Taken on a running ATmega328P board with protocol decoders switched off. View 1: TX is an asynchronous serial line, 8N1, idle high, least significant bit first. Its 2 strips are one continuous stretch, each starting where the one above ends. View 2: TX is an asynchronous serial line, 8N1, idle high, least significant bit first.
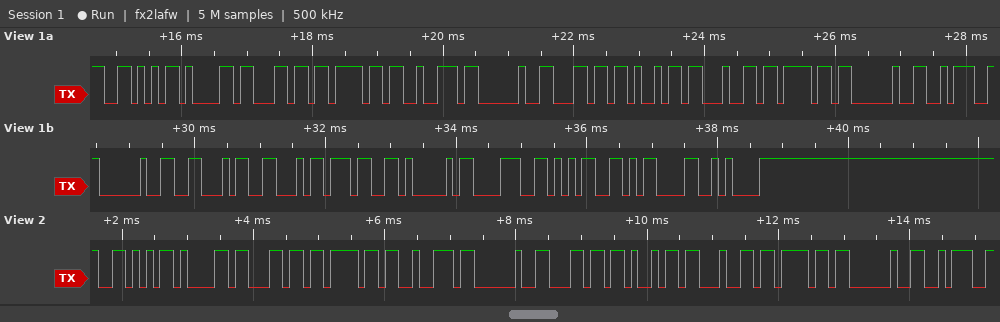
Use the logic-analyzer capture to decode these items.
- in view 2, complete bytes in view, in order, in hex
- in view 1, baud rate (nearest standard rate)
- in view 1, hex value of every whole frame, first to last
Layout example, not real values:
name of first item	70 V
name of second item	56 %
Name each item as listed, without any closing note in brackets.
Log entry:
in view 2, complete bytes in view, in order, in hex	56 61 6C 6F 72 20 6C 69 64 6F 20 3A
in view 1, baud rate	9600 baud
in view 1, hex value of every whole frame, first to last	56 61 6C 6F 72 20 6C 69 64 6F 20 3A 20 46 46 37 41 38 35 0D 0A
